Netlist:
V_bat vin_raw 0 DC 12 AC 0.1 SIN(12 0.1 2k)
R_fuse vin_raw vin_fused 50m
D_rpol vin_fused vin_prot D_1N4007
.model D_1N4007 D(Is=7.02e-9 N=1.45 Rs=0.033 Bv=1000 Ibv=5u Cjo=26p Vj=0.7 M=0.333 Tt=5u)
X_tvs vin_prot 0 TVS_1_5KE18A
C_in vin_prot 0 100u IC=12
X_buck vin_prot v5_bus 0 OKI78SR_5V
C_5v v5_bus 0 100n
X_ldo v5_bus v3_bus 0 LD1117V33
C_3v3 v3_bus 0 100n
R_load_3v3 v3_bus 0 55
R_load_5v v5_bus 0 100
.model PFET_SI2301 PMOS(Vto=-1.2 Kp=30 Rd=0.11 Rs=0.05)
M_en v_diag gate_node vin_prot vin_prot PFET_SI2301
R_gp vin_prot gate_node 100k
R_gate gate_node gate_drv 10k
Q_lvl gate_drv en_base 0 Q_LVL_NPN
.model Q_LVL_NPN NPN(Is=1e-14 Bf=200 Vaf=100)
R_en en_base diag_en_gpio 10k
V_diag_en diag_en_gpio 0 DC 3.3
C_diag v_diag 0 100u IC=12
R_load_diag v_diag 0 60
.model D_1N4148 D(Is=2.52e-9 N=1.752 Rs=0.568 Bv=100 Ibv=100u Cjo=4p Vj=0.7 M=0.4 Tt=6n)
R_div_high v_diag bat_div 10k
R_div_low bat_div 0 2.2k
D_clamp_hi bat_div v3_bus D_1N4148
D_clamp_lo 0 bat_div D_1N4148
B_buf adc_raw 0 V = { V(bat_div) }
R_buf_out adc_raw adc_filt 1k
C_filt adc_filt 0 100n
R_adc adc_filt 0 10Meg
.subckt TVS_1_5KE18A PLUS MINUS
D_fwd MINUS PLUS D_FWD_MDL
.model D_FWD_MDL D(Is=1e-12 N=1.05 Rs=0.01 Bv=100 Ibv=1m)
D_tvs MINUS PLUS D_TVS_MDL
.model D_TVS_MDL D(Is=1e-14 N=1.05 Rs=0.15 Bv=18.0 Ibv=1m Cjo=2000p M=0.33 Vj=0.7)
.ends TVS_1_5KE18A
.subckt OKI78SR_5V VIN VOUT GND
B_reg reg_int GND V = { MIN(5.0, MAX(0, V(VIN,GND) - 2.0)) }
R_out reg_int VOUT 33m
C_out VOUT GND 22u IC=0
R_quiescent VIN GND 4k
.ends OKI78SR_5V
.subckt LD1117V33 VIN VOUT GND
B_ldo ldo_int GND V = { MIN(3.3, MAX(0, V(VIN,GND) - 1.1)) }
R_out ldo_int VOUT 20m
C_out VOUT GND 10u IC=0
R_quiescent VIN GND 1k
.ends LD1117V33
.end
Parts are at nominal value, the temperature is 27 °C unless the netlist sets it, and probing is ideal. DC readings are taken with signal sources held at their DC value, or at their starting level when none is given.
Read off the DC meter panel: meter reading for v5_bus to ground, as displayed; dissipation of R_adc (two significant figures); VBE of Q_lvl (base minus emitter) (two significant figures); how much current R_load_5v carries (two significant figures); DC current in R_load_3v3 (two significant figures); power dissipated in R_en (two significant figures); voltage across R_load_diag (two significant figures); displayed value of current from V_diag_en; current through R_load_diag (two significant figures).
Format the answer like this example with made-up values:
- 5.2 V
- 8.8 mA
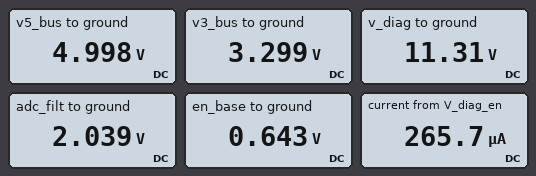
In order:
- 4.998 V
- 420 nW
- 640 mV
- 50 mA
- 60 mA
- 710 µW
- 11 V
- 265.7 µA
- 190 mA
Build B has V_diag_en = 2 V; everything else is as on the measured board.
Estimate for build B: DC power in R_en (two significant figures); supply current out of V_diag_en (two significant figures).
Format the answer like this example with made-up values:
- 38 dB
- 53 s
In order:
- 190 µW
- 140 µA
